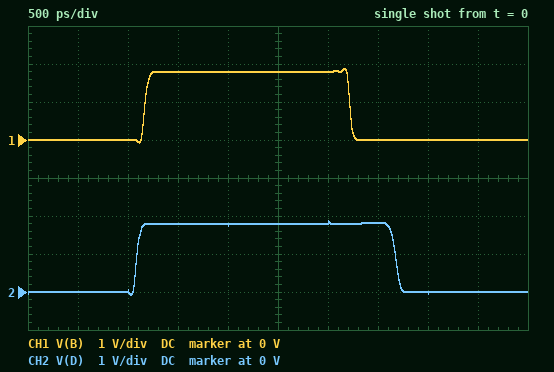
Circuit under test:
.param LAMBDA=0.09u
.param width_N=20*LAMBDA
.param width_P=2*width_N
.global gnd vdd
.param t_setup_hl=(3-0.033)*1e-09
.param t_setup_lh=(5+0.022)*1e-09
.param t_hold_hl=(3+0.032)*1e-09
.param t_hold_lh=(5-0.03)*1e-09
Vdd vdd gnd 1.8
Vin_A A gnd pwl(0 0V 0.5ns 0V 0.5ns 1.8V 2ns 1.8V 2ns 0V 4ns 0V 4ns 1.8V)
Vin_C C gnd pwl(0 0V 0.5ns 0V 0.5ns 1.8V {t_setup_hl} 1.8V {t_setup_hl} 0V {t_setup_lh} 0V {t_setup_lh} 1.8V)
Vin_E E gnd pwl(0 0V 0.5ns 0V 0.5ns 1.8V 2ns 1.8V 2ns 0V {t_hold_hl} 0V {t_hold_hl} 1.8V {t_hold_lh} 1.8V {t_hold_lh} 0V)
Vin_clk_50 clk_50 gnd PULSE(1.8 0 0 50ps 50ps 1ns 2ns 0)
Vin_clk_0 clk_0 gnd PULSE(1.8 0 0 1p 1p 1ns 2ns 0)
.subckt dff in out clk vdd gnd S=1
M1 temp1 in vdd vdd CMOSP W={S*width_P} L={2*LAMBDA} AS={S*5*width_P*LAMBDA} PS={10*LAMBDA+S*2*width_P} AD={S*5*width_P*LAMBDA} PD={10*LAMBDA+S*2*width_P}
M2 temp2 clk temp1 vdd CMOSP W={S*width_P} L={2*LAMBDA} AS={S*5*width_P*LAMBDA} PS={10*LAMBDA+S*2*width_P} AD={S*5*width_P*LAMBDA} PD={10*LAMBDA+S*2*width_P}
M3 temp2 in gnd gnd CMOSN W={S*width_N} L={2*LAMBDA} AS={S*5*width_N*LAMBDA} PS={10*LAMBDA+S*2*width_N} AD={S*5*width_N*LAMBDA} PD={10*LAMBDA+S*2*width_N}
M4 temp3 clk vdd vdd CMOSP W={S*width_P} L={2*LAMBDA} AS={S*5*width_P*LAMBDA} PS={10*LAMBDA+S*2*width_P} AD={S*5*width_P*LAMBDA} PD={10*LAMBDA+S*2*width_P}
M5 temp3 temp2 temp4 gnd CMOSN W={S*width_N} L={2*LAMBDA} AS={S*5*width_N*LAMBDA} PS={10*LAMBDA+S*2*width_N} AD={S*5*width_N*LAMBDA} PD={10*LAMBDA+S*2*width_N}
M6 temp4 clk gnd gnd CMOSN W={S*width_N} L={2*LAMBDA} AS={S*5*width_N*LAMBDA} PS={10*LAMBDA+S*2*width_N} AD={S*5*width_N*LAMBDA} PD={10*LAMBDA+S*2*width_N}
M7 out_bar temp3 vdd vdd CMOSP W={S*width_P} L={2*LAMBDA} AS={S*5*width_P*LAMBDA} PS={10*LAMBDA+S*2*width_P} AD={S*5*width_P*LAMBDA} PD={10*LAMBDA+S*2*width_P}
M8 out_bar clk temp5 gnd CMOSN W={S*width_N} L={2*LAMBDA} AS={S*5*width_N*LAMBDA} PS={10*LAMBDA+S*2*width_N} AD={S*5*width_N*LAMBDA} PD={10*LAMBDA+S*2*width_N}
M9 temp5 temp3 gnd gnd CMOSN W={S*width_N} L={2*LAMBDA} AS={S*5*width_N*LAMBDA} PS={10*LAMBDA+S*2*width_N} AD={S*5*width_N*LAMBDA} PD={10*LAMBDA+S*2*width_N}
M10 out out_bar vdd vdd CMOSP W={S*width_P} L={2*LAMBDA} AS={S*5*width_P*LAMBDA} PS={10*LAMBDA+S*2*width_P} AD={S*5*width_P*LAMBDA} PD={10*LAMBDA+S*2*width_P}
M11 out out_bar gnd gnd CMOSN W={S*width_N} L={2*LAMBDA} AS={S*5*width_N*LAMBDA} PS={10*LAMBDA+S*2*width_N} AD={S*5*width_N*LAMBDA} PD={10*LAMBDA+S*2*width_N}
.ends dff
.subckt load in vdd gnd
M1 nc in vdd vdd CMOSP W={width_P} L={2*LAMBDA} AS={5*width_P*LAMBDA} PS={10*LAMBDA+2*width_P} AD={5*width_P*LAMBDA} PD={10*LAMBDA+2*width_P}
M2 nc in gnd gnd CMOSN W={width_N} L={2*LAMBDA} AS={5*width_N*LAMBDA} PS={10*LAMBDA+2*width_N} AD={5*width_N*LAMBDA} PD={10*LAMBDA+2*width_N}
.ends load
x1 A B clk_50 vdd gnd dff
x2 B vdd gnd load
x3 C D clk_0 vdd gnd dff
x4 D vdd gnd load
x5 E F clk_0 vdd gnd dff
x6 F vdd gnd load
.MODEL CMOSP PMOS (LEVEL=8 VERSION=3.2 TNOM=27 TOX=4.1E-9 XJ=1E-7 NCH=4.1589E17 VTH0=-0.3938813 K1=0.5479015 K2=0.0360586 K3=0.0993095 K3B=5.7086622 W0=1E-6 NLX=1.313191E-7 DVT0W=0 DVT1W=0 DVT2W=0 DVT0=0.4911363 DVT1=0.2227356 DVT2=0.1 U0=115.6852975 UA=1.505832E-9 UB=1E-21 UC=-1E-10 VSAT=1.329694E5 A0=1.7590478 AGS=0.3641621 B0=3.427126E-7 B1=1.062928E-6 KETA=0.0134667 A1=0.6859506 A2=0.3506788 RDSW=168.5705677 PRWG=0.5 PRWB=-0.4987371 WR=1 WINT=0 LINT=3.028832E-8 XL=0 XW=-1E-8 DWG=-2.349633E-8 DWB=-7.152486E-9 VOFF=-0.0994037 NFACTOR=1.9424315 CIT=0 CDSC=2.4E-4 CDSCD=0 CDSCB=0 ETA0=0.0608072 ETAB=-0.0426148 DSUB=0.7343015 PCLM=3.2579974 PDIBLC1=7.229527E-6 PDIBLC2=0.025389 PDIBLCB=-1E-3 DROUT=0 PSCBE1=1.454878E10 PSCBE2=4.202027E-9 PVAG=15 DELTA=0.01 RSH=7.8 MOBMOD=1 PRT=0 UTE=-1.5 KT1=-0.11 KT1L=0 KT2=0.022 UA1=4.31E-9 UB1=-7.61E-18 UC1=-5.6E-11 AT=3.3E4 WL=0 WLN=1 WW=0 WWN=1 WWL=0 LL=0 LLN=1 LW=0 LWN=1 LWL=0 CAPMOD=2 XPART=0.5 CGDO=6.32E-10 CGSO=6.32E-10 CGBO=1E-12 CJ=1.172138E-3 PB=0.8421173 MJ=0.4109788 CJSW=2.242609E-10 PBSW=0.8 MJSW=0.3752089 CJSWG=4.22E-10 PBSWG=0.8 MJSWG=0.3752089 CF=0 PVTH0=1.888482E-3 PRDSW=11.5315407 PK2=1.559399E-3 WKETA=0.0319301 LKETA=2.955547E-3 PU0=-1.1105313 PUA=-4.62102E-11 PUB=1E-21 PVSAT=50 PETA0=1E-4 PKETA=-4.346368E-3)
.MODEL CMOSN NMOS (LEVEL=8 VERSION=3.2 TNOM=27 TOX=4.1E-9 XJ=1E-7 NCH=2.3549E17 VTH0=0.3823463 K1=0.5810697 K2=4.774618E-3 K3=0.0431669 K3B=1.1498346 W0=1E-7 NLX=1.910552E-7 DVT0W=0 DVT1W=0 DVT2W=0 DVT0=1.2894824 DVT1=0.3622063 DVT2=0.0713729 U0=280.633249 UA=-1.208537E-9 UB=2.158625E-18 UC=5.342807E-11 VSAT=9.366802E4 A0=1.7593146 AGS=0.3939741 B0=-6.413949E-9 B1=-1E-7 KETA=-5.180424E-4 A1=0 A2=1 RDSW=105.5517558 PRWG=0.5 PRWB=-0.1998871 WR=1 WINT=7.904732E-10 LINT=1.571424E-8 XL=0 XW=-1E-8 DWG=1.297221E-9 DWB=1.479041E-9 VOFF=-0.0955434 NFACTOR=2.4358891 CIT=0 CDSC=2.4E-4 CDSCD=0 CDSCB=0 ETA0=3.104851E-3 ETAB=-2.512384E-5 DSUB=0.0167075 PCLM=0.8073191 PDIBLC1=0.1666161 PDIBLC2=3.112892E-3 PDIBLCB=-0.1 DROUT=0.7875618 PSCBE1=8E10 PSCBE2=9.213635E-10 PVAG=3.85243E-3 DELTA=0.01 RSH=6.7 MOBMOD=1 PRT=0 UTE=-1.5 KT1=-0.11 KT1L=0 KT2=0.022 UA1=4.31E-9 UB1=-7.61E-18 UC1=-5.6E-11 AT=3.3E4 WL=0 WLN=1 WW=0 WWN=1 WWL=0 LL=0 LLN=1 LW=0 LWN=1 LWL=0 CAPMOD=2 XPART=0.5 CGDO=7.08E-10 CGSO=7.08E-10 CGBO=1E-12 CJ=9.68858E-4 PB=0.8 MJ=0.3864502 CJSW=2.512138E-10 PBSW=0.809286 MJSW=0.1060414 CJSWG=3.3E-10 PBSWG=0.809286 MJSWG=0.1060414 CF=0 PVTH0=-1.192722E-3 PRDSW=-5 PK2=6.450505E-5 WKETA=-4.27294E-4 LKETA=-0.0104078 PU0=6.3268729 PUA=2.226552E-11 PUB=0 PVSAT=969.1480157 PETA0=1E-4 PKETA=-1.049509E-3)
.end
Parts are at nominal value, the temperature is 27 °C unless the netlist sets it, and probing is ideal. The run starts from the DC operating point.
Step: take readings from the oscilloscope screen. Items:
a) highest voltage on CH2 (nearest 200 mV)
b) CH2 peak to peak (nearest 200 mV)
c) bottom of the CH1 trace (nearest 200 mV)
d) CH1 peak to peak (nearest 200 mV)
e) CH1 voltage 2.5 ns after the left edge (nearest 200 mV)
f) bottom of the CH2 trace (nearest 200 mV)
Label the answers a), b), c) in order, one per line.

a) 1.8 V
b) 2.0 V
c) 0 V
d) 2.0 V
e) 1.8 V
f) 0 V
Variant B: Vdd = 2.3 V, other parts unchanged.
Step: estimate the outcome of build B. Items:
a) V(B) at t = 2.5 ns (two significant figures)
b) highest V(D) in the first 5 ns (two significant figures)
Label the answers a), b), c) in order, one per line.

a) 2.3 V
b) 2.4 V
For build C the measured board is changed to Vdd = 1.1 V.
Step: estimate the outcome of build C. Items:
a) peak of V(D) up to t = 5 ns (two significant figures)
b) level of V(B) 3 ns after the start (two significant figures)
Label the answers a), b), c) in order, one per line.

a) 1.2 V
b) 1.1 V
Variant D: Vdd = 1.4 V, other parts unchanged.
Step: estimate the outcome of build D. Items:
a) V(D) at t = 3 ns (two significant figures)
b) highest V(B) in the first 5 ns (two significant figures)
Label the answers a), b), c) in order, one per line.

a) 1.4 V
b) 1.5 V
